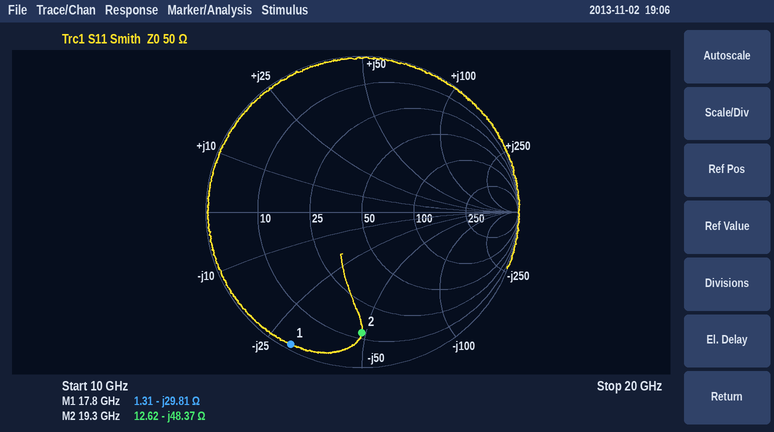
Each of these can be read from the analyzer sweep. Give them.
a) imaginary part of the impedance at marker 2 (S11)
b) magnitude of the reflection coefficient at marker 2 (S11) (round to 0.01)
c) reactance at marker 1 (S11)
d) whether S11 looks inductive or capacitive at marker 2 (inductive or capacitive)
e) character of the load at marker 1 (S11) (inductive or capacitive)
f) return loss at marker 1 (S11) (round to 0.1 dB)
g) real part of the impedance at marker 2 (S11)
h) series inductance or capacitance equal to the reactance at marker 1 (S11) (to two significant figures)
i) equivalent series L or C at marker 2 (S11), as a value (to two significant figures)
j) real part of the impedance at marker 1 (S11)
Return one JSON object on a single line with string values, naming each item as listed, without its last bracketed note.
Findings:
{"imaginary part of the impedance at marker 2": "-48.37 Ω", "magnitude of the reflection coefficient at marker 2 (S11)": "0.77", "reactance at marker 1": "-29.81 Ω", "whether S11 looks inductive or capacitive at marker 2": "capacitive", "character of the load at marker 1 (S11)": "capacitive", "return loss at marker 1 (S11)": "0.3 dB", "real part of the impedance at marker 2": "12.62 Ω", "series inductance or capacitance equal to the reactance at marker 1 (S11)": "300 fF", "equivalent series L or C at marker 2 (S11), as a value": "170 fF", "real part of the impedance at marker 1": "1.31 Ω"}
